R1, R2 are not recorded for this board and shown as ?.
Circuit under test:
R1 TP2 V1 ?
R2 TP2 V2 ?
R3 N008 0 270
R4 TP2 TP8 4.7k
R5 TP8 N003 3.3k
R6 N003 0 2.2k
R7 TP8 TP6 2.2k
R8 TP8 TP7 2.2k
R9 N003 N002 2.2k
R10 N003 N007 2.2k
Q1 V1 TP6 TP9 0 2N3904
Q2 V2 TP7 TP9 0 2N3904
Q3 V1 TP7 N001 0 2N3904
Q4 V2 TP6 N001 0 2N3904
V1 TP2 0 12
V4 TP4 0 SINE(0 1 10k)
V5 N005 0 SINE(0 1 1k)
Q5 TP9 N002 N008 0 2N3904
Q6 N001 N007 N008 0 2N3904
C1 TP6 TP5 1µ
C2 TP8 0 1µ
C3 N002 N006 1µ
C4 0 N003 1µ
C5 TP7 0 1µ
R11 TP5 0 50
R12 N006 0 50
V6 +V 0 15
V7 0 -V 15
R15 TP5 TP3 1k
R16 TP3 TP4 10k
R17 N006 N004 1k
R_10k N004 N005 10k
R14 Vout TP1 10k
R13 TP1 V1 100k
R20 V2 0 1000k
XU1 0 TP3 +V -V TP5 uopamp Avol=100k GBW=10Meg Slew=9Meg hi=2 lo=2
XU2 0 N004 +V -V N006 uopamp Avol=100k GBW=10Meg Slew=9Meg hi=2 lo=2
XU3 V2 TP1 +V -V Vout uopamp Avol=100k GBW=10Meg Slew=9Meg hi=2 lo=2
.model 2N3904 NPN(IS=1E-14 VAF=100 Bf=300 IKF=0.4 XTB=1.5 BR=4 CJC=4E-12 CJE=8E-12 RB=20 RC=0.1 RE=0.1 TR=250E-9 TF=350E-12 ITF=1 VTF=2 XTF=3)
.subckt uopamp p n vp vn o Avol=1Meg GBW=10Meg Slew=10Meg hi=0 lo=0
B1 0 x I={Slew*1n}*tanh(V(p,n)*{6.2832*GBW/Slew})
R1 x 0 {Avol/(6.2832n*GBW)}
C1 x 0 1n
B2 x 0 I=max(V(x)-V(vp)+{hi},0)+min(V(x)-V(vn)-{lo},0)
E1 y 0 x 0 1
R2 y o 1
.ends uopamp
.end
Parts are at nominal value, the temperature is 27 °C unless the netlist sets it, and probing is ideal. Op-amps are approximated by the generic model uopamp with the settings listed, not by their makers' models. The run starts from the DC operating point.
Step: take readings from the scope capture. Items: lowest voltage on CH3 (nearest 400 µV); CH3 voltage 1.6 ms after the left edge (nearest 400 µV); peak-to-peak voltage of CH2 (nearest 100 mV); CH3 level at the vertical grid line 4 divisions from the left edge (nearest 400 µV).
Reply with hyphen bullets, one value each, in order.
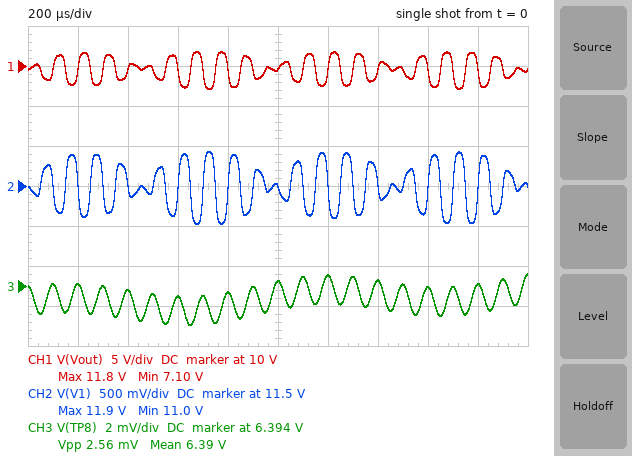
- 6.3920 V
- 6.3940 V
- 900 mV
- 6.3936 V
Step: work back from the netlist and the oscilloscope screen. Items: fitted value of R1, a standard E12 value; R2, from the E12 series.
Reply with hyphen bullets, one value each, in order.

- 150 Ω
- 680 Ω
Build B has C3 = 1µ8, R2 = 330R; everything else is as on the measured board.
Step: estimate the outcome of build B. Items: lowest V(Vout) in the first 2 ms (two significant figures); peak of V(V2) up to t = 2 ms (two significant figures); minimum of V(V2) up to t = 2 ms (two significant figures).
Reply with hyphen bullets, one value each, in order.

- 9.6 V
- 12 V
- 9.8 V
